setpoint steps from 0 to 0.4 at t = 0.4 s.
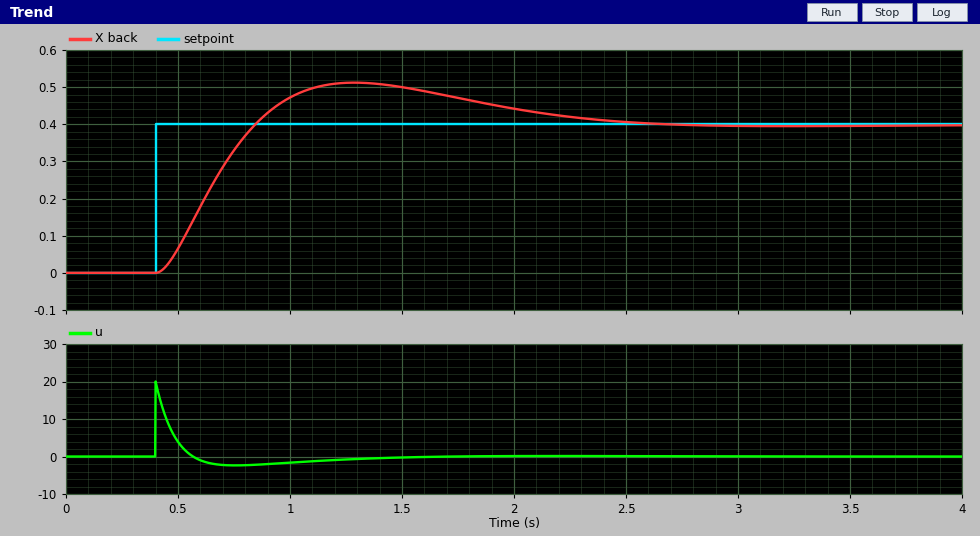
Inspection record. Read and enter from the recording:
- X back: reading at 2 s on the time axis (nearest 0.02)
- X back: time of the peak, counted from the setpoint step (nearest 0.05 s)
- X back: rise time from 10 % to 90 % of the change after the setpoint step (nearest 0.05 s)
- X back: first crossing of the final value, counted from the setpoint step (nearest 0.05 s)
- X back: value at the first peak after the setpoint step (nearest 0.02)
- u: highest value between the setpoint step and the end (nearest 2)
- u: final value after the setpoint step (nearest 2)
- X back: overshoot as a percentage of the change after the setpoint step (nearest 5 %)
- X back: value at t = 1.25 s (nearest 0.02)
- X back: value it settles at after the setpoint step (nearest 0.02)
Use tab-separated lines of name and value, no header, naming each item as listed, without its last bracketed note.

X back: reading at 2 s on the time axis	0.44
X back: time of the peak, counted from the setpoint step	0.90 s
X back: rise time from 10 % to 90 % of the change after the setpoint step	0.30 s
X back: first crossing of the final value, counted from the setpoint step	0.45 s
X back: value at the first peak after the setpoint step	0.52
u: highest value between the setpoint step and the end	20
u: final value after the setpoint step	0
X back: overshoot as a percentage of the change after the setpoint step	30 %
X back: value at t = 1.25 s	0.52
X back: value it settles at after the setpoint step	0.40
